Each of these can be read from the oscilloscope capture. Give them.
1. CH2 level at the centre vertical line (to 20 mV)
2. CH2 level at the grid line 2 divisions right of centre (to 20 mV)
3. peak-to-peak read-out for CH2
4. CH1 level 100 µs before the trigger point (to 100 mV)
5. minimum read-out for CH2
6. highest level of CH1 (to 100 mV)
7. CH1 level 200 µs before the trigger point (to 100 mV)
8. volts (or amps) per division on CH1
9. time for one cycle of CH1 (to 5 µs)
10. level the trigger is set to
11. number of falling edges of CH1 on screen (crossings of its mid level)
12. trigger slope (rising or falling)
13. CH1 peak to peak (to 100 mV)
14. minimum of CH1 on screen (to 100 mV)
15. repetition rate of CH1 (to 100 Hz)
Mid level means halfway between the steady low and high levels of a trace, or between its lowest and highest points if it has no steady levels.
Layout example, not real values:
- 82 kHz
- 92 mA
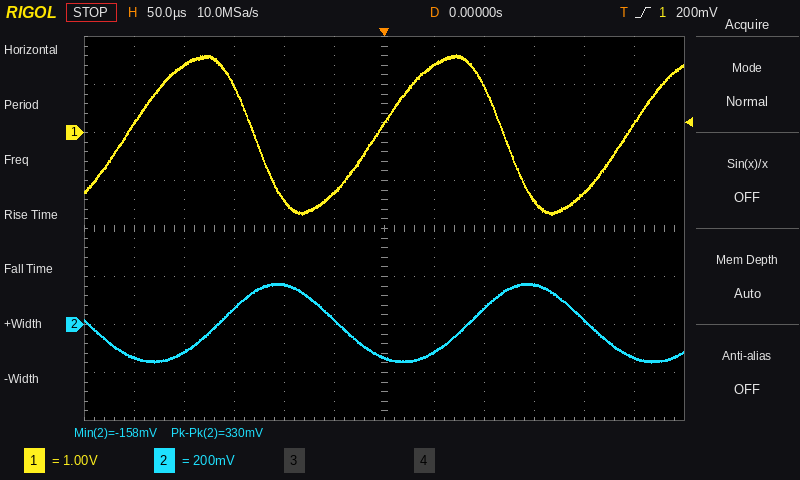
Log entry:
- -140 mV
- 60 mV
- 330 mV
- -1.4 V
- -158 mV
- 1.6 V
- 1.4 V
- 1 V
- 250 µs
- 200 mV
- 2
- rising
- 3.3 V
- -1.7 V
- 4.0 kHz
